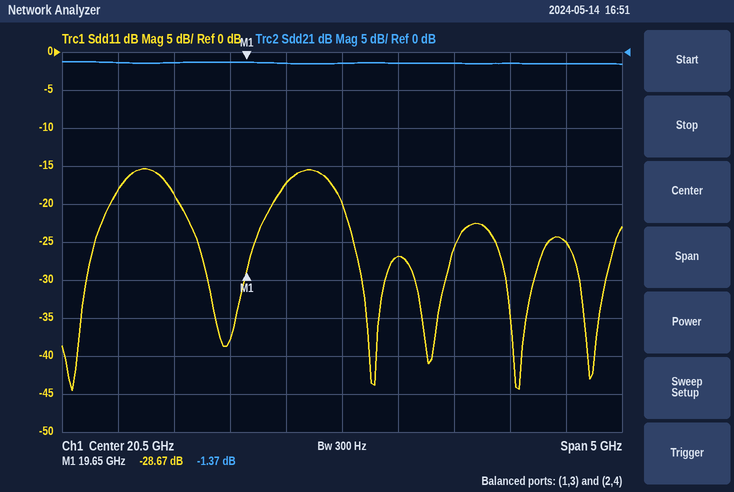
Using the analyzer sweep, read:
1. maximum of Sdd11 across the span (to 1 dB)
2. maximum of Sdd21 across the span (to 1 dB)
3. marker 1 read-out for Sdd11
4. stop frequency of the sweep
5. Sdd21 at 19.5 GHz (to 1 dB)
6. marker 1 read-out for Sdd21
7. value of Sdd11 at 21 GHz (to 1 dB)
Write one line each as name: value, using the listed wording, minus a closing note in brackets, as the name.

maximum of Sdd11 across the span: -15 dB
maximum of Sdd21 across the span: -1 dB
marker 1 read-out for Sdd11: -28.67 dB
stop frequency of the sweep: 23 GHz
Sdd21 at 19.5 GHz: -1 dB
marker 1 read-out for Sdd21: -1.37 dB
value of Sdd11 at 21 GHz: -27 dB
